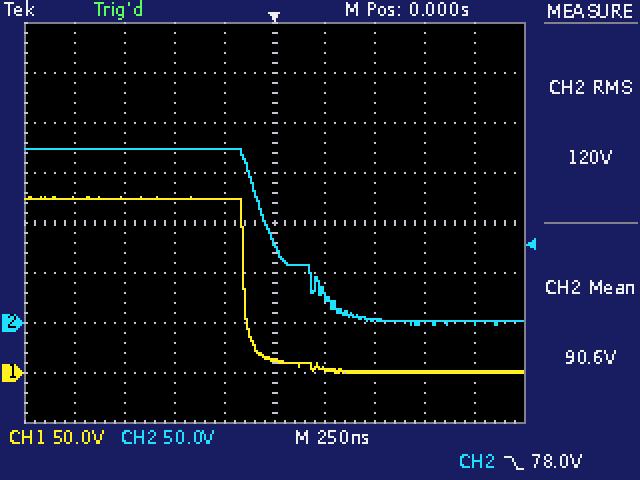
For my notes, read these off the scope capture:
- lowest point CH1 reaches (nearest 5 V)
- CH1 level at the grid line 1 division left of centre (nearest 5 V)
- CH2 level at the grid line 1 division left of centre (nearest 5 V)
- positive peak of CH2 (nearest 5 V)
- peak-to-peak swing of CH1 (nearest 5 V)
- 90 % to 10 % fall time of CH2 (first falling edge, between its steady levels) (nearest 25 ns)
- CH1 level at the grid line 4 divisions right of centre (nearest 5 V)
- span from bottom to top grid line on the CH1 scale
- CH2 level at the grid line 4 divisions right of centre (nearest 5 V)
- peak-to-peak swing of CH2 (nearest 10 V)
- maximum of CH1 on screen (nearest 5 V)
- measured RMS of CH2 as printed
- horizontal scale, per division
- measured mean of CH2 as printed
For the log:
0 V
175 V
175 V
175 V
175 V
425 ns
0 V
400 V
0 V
180 V
175 V
120 V
250 ns
90.6 V
